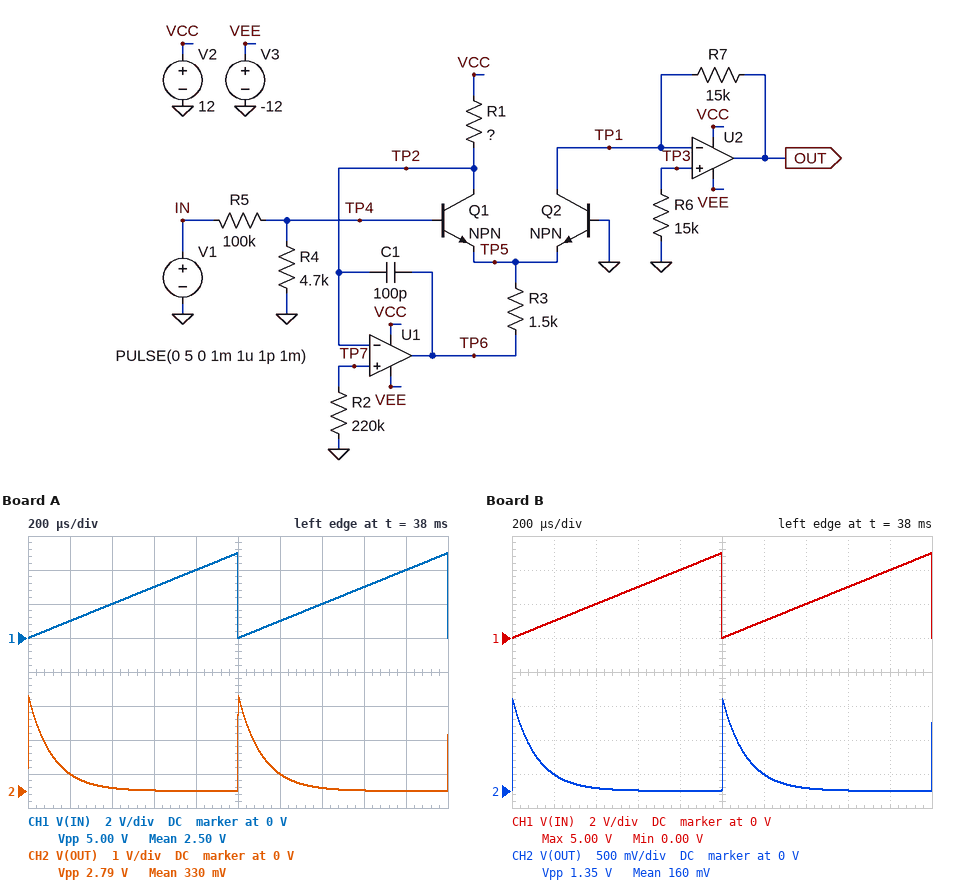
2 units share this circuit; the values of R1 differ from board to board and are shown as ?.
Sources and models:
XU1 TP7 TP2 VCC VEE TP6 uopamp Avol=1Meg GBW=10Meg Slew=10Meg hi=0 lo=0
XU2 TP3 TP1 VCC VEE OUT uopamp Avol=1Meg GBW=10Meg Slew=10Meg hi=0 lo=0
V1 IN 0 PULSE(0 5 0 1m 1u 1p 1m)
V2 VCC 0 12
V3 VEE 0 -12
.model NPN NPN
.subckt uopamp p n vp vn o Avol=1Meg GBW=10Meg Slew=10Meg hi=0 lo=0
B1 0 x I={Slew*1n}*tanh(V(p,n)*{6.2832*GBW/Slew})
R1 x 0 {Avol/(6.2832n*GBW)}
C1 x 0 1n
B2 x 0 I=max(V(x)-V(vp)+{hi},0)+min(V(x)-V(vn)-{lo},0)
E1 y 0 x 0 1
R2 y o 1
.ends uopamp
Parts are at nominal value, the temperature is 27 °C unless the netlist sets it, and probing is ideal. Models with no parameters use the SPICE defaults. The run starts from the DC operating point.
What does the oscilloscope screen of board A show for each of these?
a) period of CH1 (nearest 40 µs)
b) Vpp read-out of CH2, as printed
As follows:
1.00 ms
2.79 V
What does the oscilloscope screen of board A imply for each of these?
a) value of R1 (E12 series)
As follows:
82 kΩ
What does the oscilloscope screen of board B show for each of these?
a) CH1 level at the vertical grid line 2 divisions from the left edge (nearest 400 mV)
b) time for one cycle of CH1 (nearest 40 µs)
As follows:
2.0 V
1.00 ms
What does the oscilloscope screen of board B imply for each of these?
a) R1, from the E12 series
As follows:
150 kΩ
